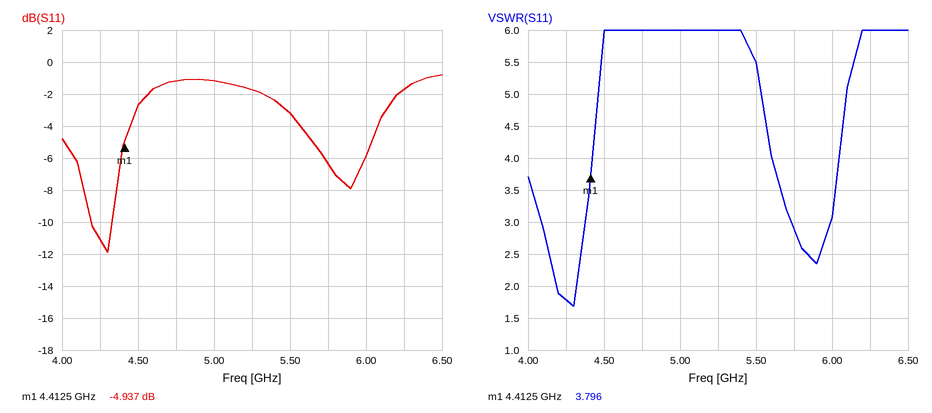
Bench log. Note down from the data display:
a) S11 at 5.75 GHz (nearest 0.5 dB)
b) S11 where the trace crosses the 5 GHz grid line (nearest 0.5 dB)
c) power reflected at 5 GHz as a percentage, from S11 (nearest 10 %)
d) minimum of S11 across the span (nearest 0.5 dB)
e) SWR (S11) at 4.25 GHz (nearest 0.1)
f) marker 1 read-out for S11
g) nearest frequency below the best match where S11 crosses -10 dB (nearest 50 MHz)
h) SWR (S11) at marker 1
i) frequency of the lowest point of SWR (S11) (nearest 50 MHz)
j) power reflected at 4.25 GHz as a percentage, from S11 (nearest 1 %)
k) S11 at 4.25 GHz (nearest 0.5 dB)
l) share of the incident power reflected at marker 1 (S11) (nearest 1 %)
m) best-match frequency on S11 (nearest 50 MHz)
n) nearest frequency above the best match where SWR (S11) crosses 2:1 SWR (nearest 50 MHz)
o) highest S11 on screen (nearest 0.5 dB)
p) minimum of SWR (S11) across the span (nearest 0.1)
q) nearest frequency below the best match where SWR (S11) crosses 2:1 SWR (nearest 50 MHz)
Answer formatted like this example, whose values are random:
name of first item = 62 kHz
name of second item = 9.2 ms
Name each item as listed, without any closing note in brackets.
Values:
S11 at 5.75 GHz = -6.5 dB
S11 where the trace crosses the 5 GHz grid line = -1.0 dB
power reflected at 5 GHz as a percentage, from S11 = 80 %
minimum of S11 across the span = -12.0 dB
SWR (S11) at 4.25 GHz = 1.8
marker 1 read-out for S11 = -4.937 dB
nearest frequency below the best match where S11 crosses -10 dB = 4.20 GHz
SWR (S11) at marker 1 = 3.796
frequency of the lowest point of SWR (S11) = 4.30 GHz
power reflected at 4.25 GHz as a percentage, from S11 = 8 %
S11 at 4.25 GHz = -11.0 dB
share of the incident power reflected at marker 1 (S11) = 32 %
best-match frequency on S11 = 4.30 GHz
nearest frequency above the best match where SWR (S11) crosses 2:1 SWR = 4.30 GHz
highest S11 on screen = -1.0 dB
minimum of SWR (S11) across the span = 1.7
nearest frequency below the best match where SWR (S11) crosses 2:1 SWR = 4.20 GHz
